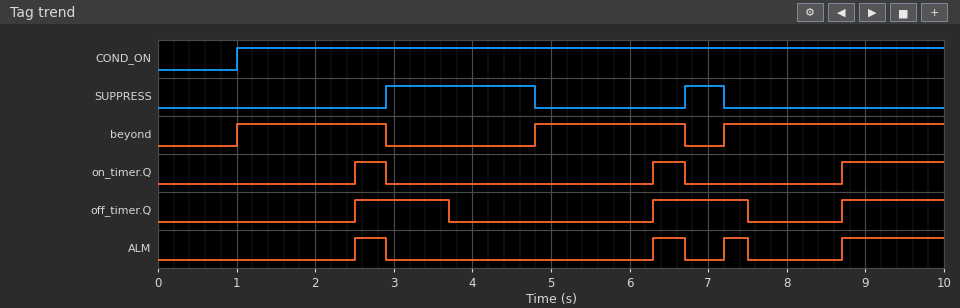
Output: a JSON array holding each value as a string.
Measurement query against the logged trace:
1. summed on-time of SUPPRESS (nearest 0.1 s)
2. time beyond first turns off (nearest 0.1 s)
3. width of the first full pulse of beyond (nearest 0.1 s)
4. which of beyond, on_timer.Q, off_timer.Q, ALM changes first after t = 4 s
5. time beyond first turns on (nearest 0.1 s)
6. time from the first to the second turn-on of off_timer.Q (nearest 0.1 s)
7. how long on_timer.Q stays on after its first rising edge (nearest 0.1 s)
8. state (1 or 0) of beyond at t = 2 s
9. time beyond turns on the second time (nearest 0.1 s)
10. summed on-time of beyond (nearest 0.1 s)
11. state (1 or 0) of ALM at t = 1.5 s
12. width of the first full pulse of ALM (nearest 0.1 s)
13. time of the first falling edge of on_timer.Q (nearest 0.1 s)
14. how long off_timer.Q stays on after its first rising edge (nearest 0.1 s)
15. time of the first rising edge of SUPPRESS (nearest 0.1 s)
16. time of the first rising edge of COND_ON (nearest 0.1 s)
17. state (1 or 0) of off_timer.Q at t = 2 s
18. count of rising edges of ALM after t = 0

["2.4 s", "2.9 s", "1.9 s", "beyond", "1.0 s", "3.8 s", "0.4 s", "1", "4.8 s", "6.6 s", "0", "0.4 s", "2.9 s", "1.2 s", "2.9 s", "1.0 s", "0", "4"]
